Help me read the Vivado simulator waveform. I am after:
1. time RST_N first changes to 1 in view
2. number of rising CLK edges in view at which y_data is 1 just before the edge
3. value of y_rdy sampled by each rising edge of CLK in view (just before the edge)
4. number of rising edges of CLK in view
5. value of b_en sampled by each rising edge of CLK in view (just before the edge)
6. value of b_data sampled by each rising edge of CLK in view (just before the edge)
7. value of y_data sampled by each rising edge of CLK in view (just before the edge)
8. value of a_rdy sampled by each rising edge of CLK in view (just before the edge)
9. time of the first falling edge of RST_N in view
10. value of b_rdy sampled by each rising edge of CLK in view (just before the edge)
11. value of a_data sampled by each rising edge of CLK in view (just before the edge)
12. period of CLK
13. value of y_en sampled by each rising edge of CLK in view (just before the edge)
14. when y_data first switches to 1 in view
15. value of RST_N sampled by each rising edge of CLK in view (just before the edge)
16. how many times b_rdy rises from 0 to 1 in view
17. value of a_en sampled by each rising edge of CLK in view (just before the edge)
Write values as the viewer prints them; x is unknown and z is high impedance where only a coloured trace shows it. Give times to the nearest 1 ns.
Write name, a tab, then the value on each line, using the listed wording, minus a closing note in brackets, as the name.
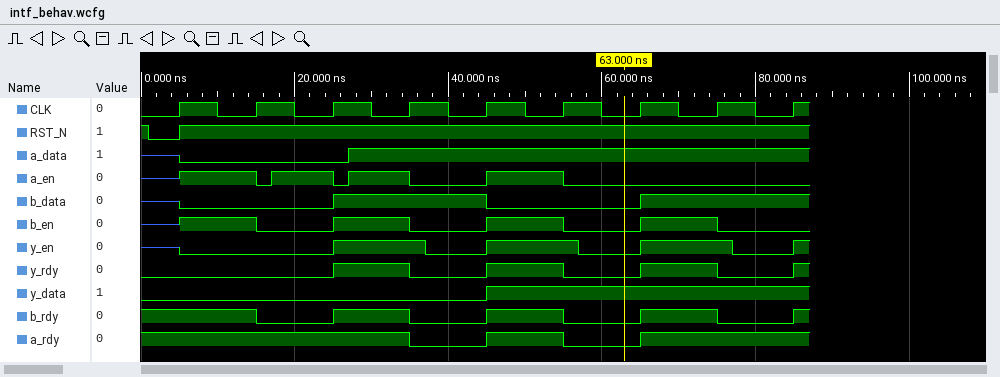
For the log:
time RST_N first changes to 1 in view	5 ns
number of rising CLK edges in view at which y_data is 1 just before the edge	4
value of y_rdy sampled by each rising edge of CLK in view	0 0 0 1 0 1 0 1 0
number of rising edges of CLK in view	9
value of b_en sampled by each rising edge of CLK in view	z 1 0 1 0 1 0 1 0
value of b_data sampled by each rising edge of CLK in view	z 0 0 1 1 0 0 1 1
value of y_data sampled by each rising edge of CLK in view	0 0 0 0 0 1 1 1 1
value of a_rdy sampled by each rising edge of CLK in view	1 1 1 1 0 1 0 1 1
time of the first falling edge of RST_N in view	1 ns
value of b_rdy sampled by each rising edge of CLK in view	1 1 0 1 0 1 0 1 0
value of a_data sampled by each rising edge of CLK in view	z 0 0 1 1 1 1 1 1
period of CLK	10 ns
value of y_en sampled by each rising edge of CLK in view	z 0 0 1 0 1 0 1 0
when y_data first switches to 1 in view	45 ns
value of RST_N sampled by each rising edge of CLK in view	0 1 1 1 1 1 1 1 1
how many times b_rdy rises from 0 to 1 in view	4
value of a_en sampled by each rising edge of CLK in view	z 1 1 1 0 1 0 0 0
